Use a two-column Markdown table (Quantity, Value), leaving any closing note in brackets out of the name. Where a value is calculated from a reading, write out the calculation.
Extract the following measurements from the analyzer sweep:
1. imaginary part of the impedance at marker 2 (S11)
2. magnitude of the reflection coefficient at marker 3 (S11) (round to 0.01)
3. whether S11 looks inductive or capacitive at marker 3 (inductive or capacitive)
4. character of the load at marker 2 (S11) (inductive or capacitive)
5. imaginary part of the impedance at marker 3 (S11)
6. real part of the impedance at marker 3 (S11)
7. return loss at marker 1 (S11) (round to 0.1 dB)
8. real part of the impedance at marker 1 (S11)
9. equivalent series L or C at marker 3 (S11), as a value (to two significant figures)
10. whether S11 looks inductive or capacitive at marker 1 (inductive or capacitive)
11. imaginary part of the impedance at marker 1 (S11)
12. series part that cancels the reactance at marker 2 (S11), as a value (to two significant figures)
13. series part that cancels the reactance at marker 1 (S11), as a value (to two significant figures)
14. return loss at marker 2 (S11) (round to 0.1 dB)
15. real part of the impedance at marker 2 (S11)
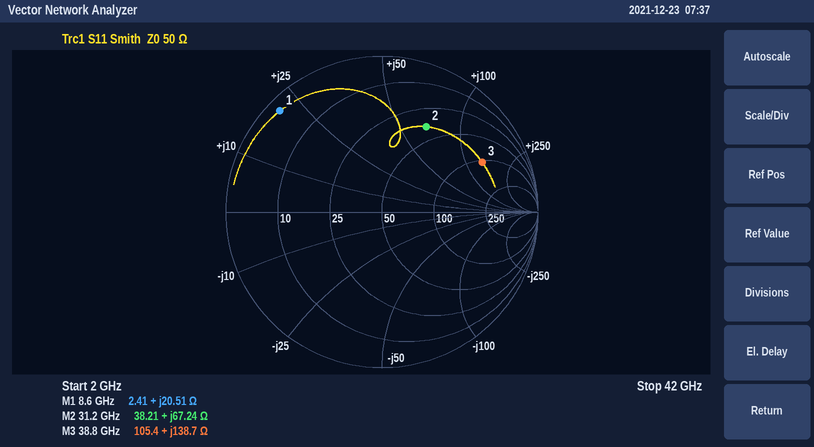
| Quantity | Value |
|---|---|
| imaginary part of the impedance at marker 2 | +67.24 Ω |
| magnitude of the reflection coefficient at marker 3 (S11) | 0.72 |
| whether S11 looks inductive or capacitive at marker 3 | inductive |
| character of the load at marker 2 (S11) | inductive |
| imaginary part of the impedance at marker 3 | +138.7 Ω |
| real part of the impedance at marker 3 | 105.4 Ω |
| return loss at marker 1 (S11) | 0.7 dB |
| real part of the impedance at marker 1 | 2.41 Ω |
| equivalent series L or C at marker 3 (S11), as a value | L = 138.7 Ω/(2π × 38.8 GHz) ≈ 569 pH, so 570 pH to two significant figures |
| whether S11 looks inductive or capacitive at marker 1 | inductive |
| imaginary part of the impedance at marker 1 | +20.51 Ω |
| series part that cancels the reactance at marker 2 (S11), as a value | C = 1/(2π × 31.2 GHz × 67.24 Ω) ≈ 76 fF |
| series part that cancels the reactance at marker 1 (S11), as a value | C = 1/(2π × 8.6 GHz × 20.51 Ω) ≈ 902 fF, so 900 fF to two significant figures |
| return loss at marker 2 (S11) | 4.2 dB |
| real part of the impedance at marker 2 | 38.21 Ω |
